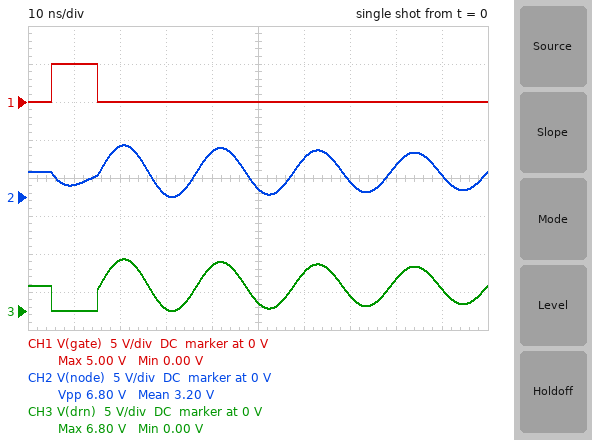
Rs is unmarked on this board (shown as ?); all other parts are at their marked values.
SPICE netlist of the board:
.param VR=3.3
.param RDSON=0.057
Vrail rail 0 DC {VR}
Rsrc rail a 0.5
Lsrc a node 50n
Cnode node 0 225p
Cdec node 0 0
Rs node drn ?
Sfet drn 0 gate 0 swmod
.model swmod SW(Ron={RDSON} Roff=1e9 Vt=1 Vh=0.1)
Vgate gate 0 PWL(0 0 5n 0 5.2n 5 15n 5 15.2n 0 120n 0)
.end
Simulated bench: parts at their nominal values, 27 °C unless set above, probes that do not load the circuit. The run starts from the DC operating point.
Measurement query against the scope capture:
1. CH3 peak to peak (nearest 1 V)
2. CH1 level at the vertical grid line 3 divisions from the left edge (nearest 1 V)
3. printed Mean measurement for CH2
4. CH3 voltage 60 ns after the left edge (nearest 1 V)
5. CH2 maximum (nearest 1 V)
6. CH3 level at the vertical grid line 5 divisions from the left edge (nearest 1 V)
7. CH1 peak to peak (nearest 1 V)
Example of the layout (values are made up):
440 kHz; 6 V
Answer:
7 V; 0 V; 3.20 V; 5 V; 7 V; 1 V; 5 V
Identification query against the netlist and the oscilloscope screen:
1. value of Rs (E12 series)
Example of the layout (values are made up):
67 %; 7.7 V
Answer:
15 Ω
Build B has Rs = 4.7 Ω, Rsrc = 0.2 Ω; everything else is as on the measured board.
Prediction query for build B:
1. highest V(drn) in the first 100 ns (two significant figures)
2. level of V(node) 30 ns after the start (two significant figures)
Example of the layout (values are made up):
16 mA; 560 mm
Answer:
9.6 V; -2.1 V
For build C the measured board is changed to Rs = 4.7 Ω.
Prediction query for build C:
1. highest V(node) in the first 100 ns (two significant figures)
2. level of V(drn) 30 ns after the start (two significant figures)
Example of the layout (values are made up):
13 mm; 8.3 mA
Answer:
9.4 V; -1.7 V
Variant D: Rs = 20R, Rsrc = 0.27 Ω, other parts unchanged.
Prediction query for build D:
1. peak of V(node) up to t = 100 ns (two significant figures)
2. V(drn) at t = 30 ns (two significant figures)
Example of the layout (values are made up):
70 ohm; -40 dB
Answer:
6.3 V; 590 mV
